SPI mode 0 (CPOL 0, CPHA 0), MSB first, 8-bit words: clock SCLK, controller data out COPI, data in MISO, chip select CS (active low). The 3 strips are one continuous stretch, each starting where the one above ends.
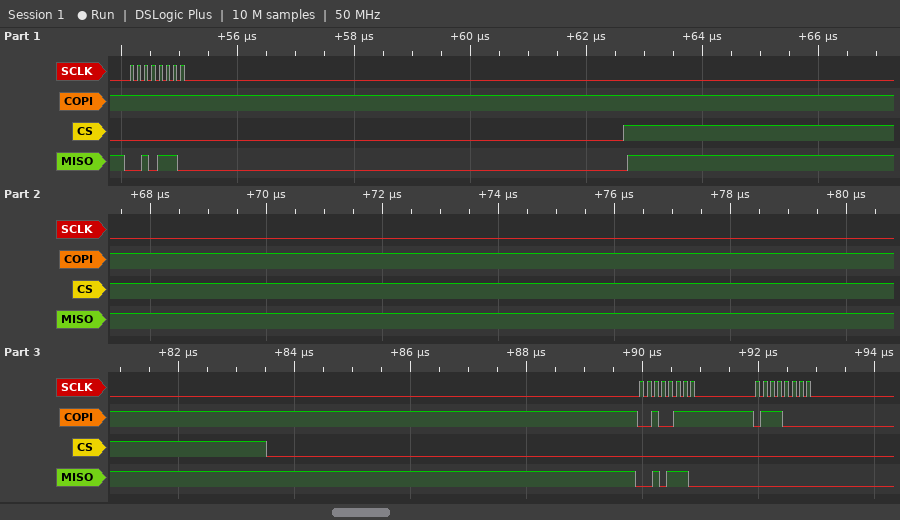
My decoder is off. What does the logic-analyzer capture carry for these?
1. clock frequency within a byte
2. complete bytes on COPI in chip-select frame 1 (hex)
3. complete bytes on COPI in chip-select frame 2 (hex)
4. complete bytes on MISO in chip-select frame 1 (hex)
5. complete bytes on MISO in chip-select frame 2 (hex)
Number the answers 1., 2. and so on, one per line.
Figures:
1. 8 MHz
2. 0xFF
3. 0x27 0x70
4. 0x2E
5. 0x2E 0x00
